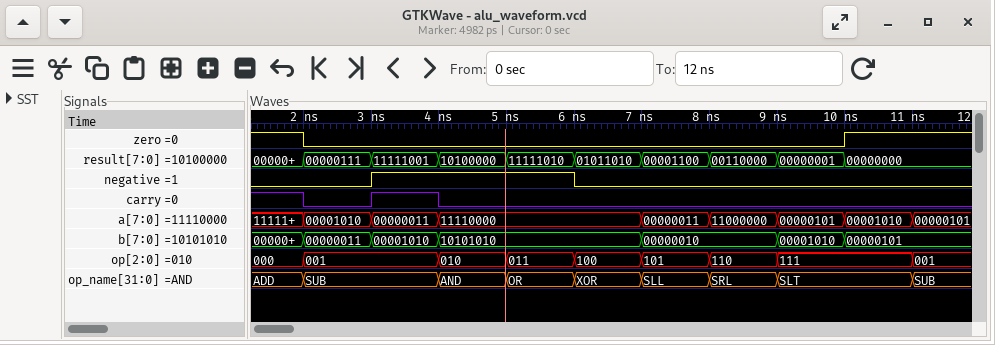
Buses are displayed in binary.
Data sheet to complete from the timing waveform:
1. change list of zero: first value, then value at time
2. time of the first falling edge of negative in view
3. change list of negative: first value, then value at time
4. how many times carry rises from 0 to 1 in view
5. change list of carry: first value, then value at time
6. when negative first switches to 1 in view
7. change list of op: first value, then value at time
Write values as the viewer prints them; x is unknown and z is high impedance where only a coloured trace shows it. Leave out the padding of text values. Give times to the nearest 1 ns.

1, 0 at 2 ns, 1 at 10 ns
6 ns
0, 1 at 3 ns, 0 at 6 ns
1
1, 0 at 2 ns, 1 at 3 ns, 0 at 4 ns
3 ns
000, 001 at 2 ns, 010 at 4 ns, 011 at 5 ns, 100 at 6 ns, 101 at 7 ns, 110 at 8 ns, 111 at 9 ns, 001 at 11 ns
